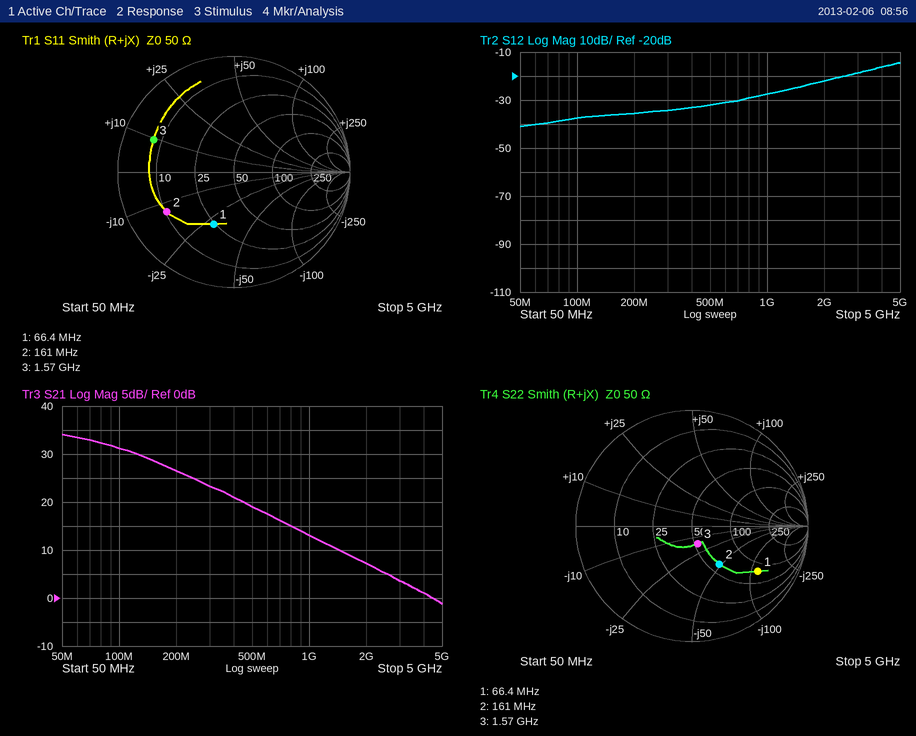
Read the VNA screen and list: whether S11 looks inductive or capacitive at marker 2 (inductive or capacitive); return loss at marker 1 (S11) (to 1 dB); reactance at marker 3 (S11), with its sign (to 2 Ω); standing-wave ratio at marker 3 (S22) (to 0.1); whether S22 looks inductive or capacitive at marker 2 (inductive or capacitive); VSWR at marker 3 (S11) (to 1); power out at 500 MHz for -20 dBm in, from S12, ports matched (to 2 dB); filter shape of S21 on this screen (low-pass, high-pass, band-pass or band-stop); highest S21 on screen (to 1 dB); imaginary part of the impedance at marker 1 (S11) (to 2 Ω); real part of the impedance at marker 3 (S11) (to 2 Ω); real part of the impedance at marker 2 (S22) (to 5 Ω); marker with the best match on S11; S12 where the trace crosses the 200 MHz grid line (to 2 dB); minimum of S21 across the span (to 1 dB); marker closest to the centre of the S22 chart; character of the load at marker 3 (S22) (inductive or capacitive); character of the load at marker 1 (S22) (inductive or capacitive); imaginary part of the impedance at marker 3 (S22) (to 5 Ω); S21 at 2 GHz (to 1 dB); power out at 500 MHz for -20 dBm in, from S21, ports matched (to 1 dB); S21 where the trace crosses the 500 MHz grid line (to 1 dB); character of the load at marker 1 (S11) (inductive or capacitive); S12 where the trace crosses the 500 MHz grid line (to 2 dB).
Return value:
capacitive
6 dB
+10 Ω
1.4
capacitive
7
-52 dBm
low-pass
34 dB
-28 Ω
8 Ω
60 Ω
marker 1
-36 dB
-1 dB
marker 3
capacitive
capacitive
-15 Ω
7 dB
-1 dBm
19 dB
capacitive
-32 dB
